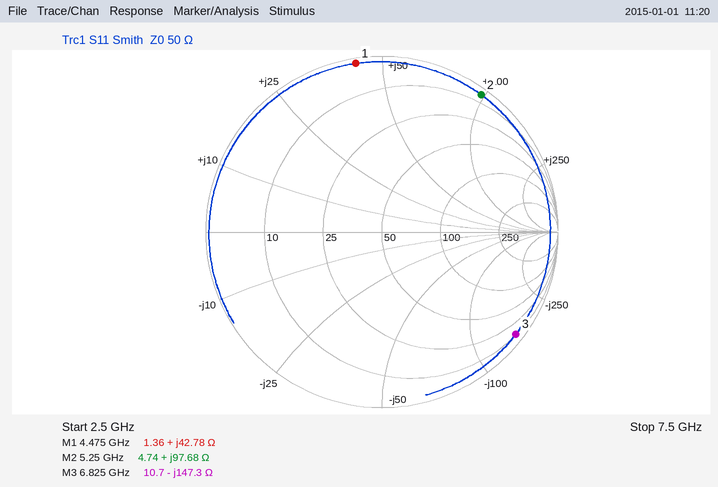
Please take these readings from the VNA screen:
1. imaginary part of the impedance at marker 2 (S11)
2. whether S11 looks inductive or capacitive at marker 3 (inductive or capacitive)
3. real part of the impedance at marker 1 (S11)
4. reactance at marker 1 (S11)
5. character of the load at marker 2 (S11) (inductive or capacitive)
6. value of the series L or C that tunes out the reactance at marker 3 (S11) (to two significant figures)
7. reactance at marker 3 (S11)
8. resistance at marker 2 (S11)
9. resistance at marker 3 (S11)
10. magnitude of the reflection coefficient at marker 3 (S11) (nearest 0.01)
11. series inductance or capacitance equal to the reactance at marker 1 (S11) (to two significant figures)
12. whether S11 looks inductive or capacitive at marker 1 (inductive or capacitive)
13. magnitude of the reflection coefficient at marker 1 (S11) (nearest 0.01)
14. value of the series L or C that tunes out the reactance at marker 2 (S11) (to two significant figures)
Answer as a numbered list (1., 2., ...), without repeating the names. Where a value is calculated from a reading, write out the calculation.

1. +97.68 Ω
2. capacitive
3. 1.36 Ω
4. +42.78 Ω
5. inductive
6. L = 147.3 Ω/(2π × 6.825 GHz) ≈ 3.4 nH
7. -147.3 Ω
8. 4.74 Ω
9. 10.7 Ω
10. 0.96
11. L = 42.78 Ω/(2π × 4.475 GHz) ≈ 1.5 nH
12. inductive
13. 0.97
14. C = 1/(2π × 5.25 GHz × 97.68 Ω) ≈ 310 fF
